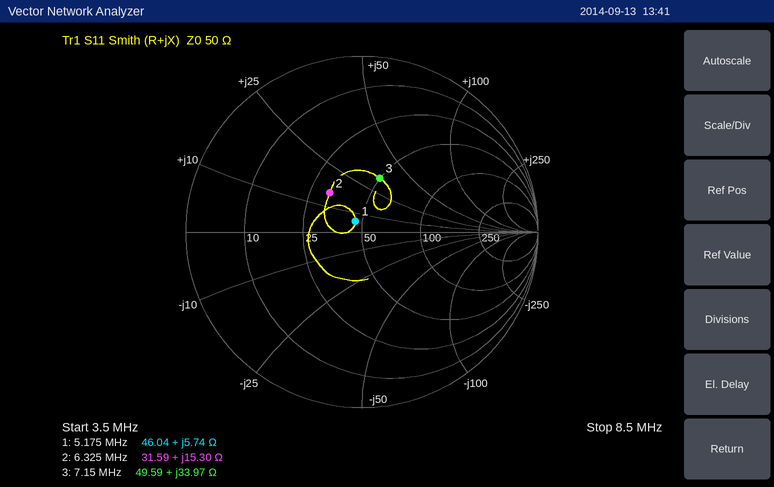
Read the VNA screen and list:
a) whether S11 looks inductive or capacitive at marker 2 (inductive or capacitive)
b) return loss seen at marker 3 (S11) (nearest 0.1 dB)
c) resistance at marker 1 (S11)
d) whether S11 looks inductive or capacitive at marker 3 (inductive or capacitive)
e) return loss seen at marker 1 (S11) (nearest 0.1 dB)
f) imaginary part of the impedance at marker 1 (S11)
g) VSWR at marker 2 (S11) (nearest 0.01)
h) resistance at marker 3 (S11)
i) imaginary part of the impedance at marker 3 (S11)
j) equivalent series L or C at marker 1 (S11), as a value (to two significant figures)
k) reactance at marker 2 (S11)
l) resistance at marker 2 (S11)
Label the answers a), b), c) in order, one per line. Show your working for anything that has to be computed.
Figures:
a) inductive
b) 9.8 dB
c) 46.04 Ω
d) inductive
e) 22.8 dB
f) +5.74 Ω
g) 1.81
h) 49.59 Ω
i) +33.97 Ω
j) L = 5.74 Ω/(2π × 5.175 MHz) ≈ 177 nH, so 180 nH to two significant figures
k) +15.30 Ω
l) 31.59 Ω
